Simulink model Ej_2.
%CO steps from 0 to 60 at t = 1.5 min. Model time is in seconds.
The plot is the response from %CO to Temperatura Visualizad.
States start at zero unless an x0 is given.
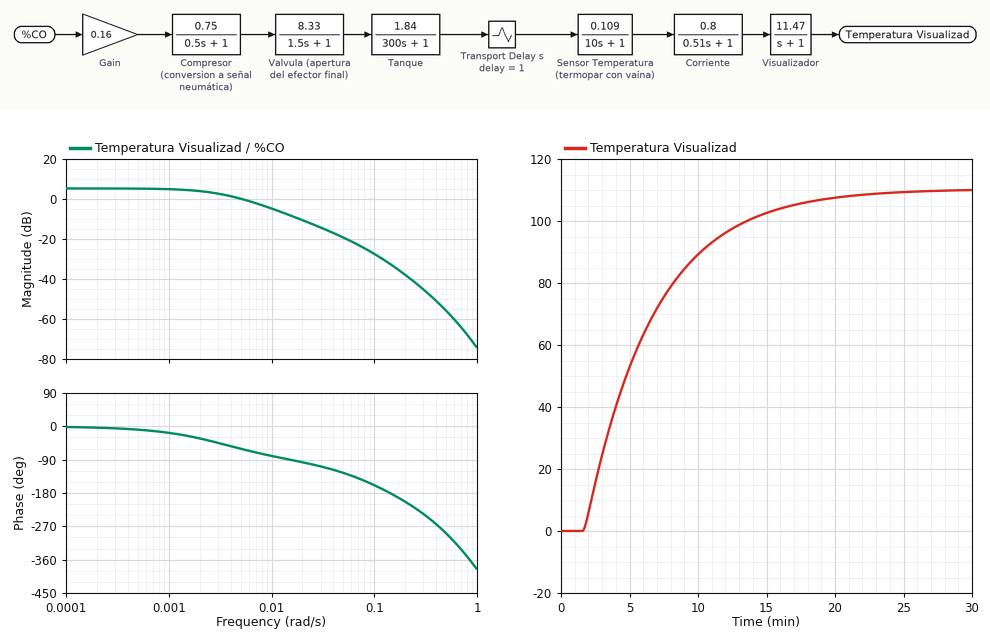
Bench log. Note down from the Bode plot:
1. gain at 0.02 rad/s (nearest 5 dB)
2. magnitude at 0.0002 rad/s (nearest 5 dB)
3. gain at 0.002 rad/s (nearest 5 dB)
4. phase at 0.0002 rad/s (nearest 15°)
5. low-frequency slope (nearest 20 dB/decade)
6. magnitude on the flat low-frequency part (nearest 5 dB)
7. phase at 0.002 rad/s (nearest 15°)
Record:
-10 dB
5 dB
5 dB
0°
0 dB/decade
5 dB
-30°
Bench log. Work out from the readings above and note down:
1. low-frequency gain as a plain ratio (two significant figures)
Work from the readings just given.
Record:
1.8
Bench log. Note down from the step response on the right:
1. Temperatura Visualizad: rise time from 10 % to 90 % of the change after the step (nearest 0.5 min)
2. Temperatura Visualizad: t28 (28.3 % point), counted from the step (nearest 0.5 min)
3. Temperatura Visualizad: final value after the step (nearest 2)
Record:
11.0 min
2.0 min
110
